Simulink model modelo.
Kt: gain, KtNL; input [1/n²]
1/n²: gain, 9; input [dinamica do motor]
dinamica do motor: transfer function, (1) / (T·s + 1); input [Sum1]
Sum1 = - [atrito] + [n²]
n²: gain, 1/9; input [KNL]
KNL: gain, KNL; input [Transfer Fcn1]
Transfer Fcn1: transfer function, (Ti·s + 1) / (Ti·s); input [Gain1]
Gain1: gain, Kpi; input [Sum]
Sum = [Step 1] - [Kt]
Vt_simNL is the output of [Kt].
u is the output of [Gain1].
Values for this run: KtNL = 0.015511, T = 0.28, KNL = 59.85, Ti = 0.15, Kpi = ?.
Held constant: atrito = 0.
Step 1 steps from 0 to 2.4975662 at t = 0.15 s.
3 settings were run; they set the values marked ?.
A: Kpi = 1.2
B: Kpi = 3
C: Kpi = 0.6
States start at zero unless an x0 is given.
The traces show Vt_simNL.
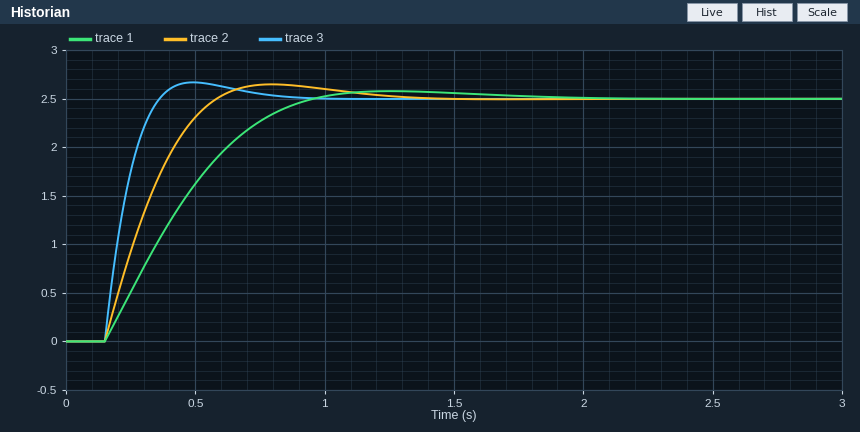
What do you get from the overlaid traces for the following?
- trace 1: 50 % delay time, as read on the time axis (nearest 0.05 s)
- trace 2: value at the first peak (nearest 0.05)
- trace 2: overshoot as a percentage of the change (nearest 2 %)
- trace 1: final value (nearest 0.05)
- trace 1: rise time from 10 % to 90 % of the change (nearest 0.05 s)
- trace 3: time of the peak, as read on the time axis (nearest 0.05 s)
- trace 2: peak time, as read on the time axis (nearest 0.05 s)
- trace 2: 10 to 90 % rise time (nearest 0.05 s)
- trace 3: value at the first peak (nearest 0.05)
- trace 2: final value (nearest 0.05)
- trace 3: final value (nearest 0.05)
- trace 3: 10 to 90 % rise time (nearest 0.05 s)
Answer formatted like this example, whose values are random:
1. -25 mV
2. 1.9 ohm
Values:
1. 0.40 s
2. 2.65
3. 6 %
4. 2.50
5. 0.55 s
6. 0.50 s
7. 0.80 s
8. 0.30 s
9. 2.65
10. 2.50
11. 2.50
12. 0.15 s
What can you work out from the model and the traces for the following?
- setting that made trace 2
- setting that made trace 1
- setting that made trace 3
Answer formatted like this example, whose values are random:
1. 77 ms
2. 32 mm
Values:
1. A
2. C
3. B
